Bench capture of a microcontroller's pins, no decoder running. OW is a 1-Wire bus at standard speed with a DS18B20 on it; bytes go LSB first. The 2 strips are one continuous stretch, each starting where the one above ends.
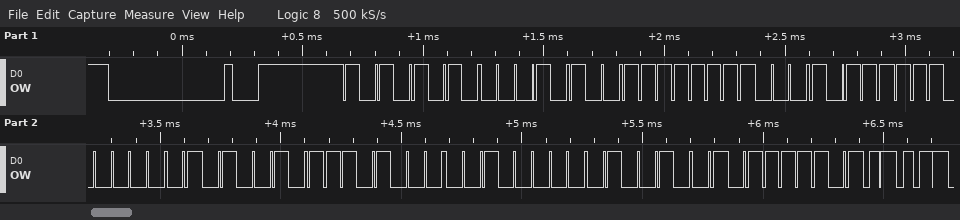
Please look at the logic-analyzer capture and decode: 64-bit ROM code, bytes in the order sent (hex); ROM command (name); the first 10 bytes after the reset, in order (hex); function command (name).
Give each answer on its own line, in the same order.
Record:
28 FF E8 07 4A 17 04 92
Match ROM
55 28 FF E8 07 4A 17 04 92 BE
Read Scratchpad
